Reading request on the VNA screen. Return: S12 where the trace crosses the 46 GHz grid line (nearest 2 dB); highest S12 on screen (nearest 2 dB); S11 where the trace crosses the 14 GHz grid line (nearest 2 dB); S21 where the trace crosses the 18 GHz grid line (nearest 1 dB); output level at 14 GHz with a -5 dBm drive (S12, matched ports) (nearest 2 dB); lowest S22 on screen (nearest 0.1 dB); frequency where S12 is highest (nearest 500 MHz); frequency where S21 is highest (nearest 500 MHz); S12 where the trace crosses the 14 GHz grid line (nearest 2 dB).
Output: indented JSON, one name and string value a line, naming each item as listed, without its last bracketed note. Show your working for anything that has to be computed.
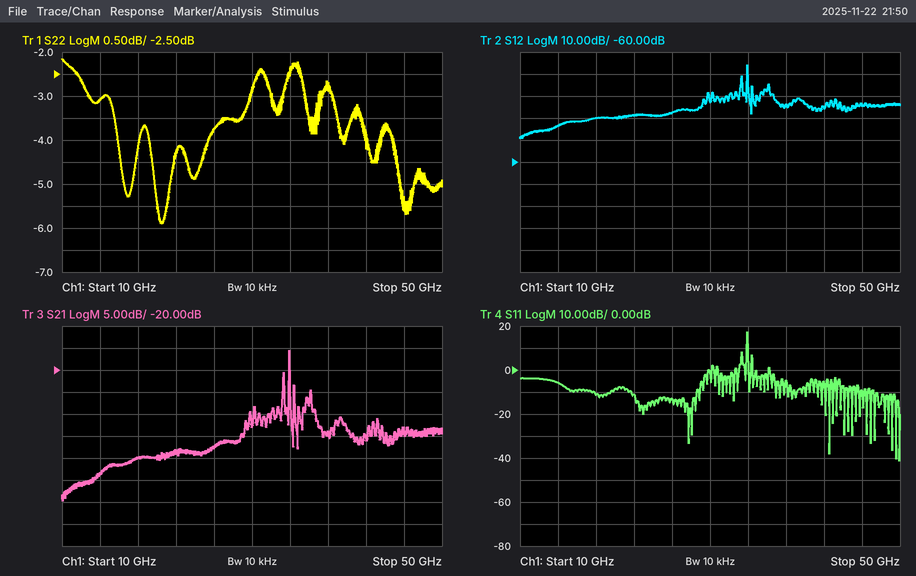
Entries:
{
  "S12 where the trace crosses the 46 GHz grid line": "-34 dB",
  "highest S12 on screen": "-16 dB",
  "S11 where the trace crosses the 14 GHz grid line": "-6 dB",
  "S21 where the trace crosses the 18 GHz grid line": "-40 dB",
  "output level at 14 GHz with a -5 dBm drive (S12, matched ports)": "-5 dBm + (-44 dB) = -48 dBm",
  "lowest S22 on screen": "-5.9 dB",
  "frequency where S12 is highest": "34.0 GHz",
  "frequency where S21 is highest": "34.0 GHz",
  "S12 where the trace crosses the 14 GHz grid line": "-44 dB"
}
